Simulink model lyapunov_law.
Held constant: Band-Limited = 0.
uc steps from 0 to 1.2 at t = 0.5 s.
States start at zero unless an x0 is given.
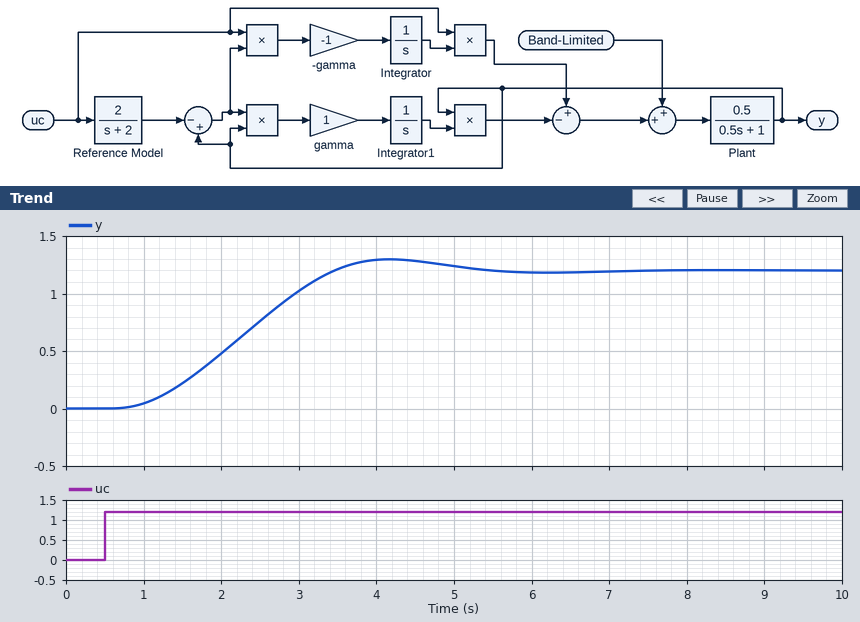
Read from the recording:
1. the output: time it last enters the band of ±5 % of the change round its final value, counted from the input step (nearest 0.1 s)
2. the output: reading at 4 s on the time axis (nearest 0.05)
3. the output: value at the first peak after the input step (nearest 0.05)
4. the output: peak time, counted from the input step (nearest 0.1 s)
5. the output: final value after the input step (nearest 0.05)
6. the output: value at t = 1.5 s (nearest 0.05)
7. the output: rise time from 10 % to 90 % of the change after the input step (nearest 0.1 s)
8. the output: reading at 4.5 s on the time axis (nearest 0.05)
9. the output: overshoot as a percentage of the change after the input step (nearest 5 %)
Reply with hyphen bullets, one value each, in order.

- 4.3 s
- 1.30
- 1.30
- 3.7 s
- 1.20
- 0.20
- 1.9 s
- 1.30
- 10 %
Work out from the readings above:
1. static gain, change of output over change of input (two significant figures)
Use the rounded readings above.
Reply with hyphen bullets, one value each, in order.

- 1.0
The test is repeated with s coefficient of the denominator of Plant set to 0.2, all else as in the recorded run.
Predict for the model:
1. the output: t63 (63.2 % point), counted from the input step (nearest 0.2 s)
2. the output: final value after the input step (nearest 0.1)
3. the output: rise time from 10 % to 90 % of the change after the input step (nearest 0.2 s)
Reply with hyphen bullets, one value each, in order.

- 1.8 s
- 1.2
- 2.0 s
